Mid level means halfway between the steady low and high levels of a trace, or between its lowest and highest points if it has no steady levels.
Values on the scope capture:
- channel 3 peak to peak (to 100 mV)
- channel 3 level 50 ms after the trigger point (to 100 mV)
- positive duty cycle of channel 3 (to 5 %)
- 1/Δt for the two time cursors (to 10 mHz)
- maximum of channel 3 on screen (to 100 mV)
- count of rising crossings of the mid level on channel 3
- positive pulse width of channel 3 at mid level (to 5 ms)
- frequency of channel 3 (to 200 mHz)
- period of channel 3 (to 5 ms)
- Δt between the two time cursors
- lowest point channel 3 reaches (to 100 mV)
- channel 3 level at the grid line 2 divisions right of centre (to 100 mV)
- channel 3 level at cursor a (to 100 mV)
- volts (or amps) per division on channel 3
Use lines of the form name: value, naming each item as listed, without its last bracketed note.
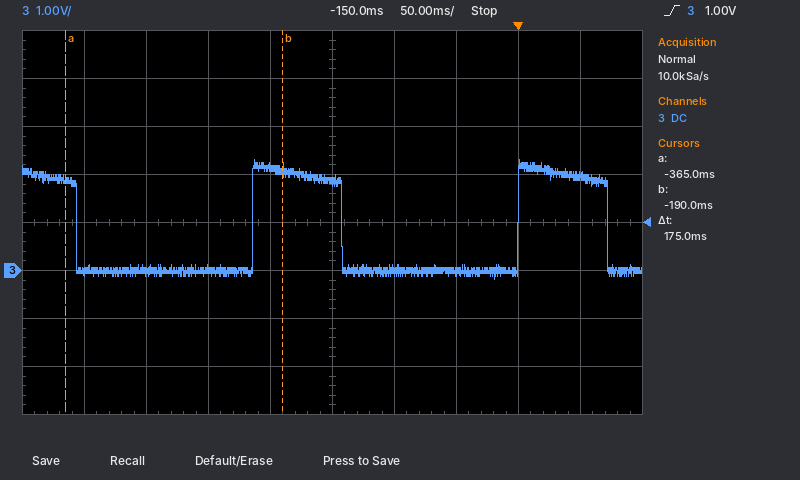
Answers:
channel 3 peak to peak: 2.5 V
channel 3 level 50 ms after the trigger point: 2.0 V
positive duty cycle of channel 3: 35 %
1/Δt for the two time cursors: 5.71 Hz
maximum of channel 3 on screen: 2.3 V
count of rising crossings of the mid level on channel 3: 2
positive pulse width of channel 3 at mid level: 70 ms
frequency of channel 3: 4.6 Hz
period of channel 3: 215 ms
Δt between the two time cursors: 175 ms
lowest point channel 3 reaches: -200 mV
channel 3 level at the grid line 2 divisions right of centre: 0.0 V
channel 3 level at cursor a: 1.9 V
volts (or amps) per division on channel 3: 1 V
